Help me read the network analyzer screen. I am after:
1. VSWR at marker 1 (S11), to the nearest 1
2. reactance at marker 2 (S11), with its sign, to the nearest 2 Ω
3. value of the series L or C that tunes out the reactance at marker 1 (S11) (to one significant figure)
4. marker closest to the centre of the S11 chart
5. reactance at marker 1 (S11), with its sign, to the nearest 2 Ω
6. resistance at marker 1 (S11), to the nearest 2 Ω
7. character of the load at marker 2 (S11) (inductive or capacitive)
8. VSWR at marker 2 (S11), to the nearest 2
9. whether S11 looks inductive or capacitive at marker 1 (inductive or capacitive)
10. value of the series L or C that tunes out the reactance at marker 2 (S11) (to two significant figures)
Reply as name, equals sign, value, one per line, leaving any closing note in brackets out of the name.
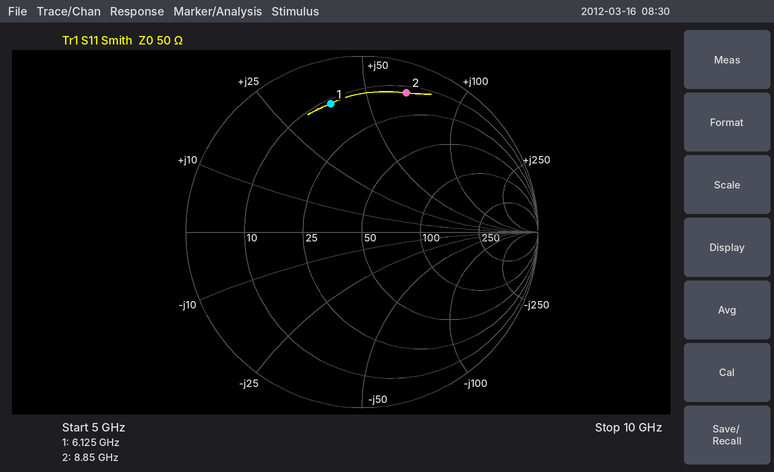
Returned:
VSWR at marker 1 (S11), to the nearest 1 = 7
reactance at marker 2 (S11), with its sign, to the nearest 2 Ω = +66 Ω
value of the series L or C that tunes out the reactance at marker 1 (S11) = 700 fF
marker closest to the centre of the S11 chart = marker 1
reactance at marker 1 (S11), with its sign, to the nearest 2 Ω = +38 Ω
resistance at marker 1 (S11), to the nearest 2 Ω = 12 Ω
character of the load at marker 2 (S11) = inductive
VSWR at marker 2 (S11), to the nearest 2 = 10
whether S11 looks inductive or capacitive at marker 1 = inductive
value of the series L or C that tunes out the reactance at marker 2 (S11) = 270 fF
